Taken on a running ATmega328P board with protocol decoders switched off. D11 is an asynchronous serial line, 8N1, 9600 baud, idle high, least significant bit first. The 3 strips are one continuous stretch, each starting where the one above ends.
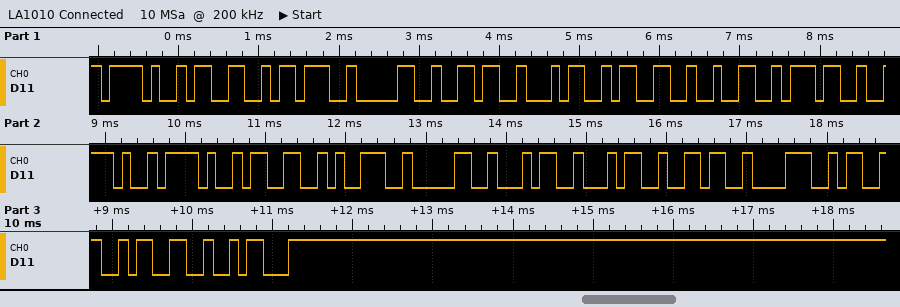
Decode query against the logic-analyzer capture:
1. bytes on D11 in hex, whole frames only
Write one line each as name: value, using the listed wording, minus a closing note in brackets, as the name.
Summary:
bytes on D11 in hex, whole frames only: 0x2F 0x33 0x3B 0x30 0x36 0x34 0x33 0x32 0x37 0x2E 0x2F 0x33 0x39 0x30 0x34 0x34 0x36 0x38 0x33 0x33 0x1A
